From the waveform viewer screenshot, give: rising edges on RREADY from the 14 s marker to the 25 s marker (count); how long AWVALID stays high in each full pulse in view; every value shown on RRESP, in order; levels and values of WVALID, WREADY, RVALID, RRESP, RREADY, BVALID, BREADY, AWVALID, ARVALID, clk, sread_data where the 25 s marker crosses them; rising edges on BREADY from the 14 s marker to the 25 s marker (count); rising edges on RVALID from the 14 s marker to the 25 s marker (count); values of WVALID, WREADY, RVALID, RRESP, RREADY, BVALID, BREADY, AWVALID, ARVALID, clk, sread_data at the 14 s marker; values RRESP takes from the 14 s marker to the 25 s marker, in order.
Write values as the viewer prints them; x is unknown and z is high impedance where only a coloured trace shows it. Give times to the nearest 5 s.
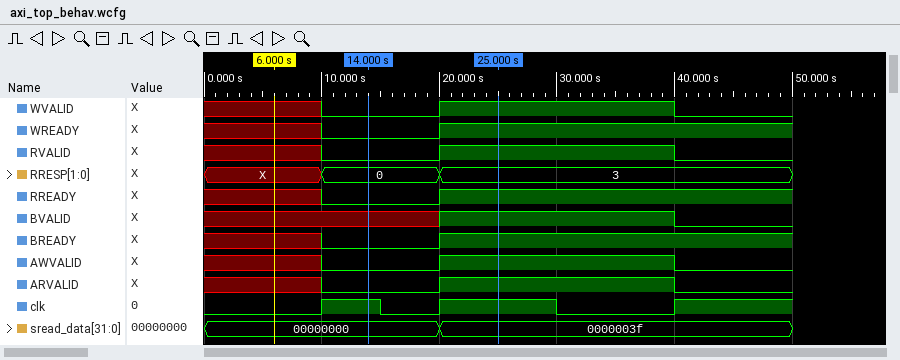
1
20 s
X, 0, 3
WVALID=1, WREADY=1, RVALID=1, RRESP=3, RREADY=1, BVALID=1, BREADY=1, AWVALID=1, ARVALID=1, clk=1, sread_data=0000003f
1
1
WVALID=0, WREADY=0, RVALID=0, RRESP=0, RREADY=0, BVALID=x, BREADY=0, AWVALID=0, ARVALID=0, clk=1, sread_data=00000000
0, 3
